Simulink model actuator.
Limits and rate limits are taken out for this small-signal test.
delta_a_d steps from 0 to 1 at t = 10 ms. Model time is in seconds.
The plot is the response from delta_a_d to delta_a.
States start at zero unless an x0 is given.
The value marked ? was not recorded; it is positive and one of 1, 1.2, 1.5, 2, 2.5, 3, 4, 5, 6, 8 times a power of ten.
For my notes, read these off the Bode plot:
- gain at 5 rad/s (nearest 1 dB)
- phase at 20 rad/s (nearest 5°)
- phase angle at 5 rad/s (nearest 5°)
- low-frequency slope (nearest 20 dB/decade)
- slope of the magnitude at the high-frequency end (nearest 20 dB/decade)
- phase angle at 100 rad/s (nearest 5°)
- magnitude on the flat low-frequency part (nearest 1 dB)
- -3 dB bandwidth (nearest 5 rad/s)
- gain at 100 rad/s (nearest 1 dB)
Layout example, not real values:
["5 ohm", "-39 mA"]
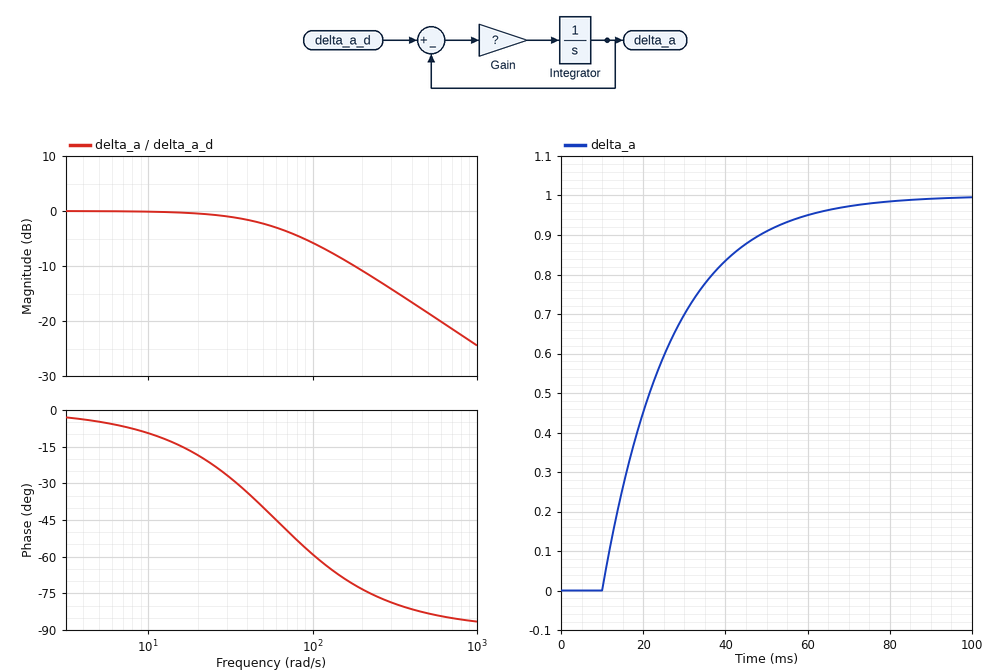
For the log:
["0 dB", "-20°", "-5°", "0 dB/decade", "-20 dB/decade", "-60°", "0 dB", "60 rad/s", "-6 dB"]
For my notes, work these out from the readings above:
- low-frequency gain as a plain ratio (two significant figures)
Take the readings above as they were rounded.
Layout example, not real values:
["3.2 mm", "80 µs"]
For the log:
["1.0"]
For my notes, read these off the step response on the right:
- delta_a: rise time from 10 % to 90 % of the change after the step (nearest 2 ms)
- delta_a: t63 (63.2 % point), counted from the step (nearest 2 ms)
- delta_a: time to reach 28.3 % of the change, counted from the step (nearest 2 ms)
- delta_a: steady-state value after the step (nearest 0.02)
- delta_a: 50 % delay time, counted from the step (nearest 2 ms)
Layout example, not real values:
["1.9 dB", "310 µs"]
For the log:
["36 ms", "16 ms", "6 ms", "1.00", "12 ms"]
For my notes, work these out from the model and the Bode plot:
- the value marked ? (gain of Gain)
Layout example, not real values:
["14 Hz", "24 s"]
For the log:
["60"]
